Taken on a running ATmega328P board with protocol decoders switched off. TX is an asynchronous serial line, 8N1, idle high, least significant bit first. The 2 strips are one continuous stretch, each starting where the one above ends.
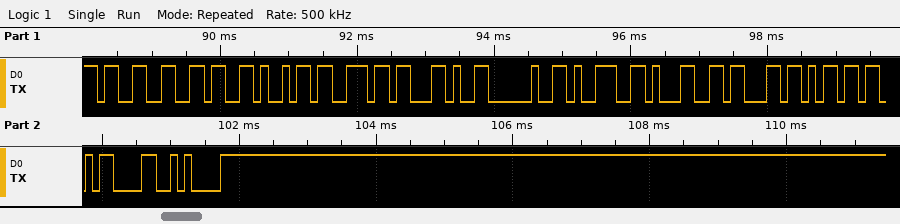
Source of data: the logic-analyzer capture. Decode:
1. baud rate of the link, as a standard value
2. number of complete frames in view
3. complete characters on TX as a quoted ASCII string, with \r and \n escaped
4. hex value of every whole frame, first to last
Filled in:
9600 baud
12
"36in, 91cm\r\n"
33 36 69 6E 2C 20 39 31 63 6D 0D 0A
